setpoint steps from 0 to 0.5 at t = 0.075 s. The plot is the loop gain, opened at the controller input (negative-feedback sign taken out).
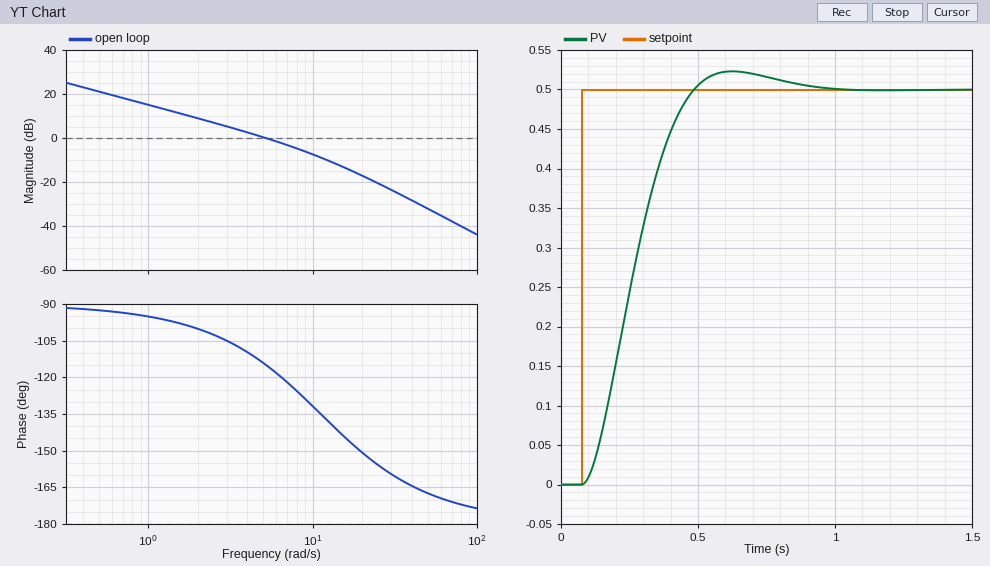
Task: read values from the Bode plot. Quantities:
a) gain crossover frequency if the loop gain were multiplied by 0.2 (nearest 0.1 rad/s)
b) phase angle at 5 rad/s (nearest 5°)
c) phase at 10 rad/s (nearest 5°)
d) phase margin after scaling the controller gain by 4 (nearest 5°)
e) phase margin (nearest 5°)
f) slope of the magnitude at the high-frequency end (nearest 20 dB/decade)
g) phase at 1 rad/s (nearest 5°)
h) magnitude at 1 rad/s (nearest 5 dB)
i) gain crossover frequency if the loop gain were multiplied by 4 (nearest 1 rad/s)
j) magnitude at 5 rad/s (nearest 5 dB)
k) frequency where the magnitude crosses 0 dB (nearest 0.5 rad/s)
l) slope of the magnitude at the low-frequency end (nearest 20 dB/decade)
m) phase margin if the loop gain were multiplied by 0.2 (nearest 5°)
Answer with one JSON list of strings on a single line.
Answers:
["1.1 rad/s", "-115°", "-130°", "40°", "65°", "-40 dB/decade", "-95°", "15 dB", "14 rad/s", "0 dB", "5.0 rad/s", "-20 dB/decade", "85°"]
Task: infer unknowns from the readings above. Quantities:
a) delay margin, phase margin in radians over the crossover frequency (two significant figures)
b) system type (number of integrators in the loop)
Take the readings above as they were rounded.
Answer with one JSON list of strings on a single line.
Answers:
["0.23 s", "1"]
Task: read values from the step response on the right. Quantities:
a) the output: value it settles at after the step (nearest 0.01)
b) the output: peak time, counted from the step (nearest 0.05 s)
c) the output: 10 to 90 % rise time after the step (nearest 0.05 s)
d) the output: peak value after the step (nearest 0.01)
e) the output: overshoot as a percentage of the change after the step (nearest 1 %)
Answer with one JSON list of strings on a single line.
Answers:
["0.50", "0.55 s", "0.25 s", "0.52", "5 %"]
